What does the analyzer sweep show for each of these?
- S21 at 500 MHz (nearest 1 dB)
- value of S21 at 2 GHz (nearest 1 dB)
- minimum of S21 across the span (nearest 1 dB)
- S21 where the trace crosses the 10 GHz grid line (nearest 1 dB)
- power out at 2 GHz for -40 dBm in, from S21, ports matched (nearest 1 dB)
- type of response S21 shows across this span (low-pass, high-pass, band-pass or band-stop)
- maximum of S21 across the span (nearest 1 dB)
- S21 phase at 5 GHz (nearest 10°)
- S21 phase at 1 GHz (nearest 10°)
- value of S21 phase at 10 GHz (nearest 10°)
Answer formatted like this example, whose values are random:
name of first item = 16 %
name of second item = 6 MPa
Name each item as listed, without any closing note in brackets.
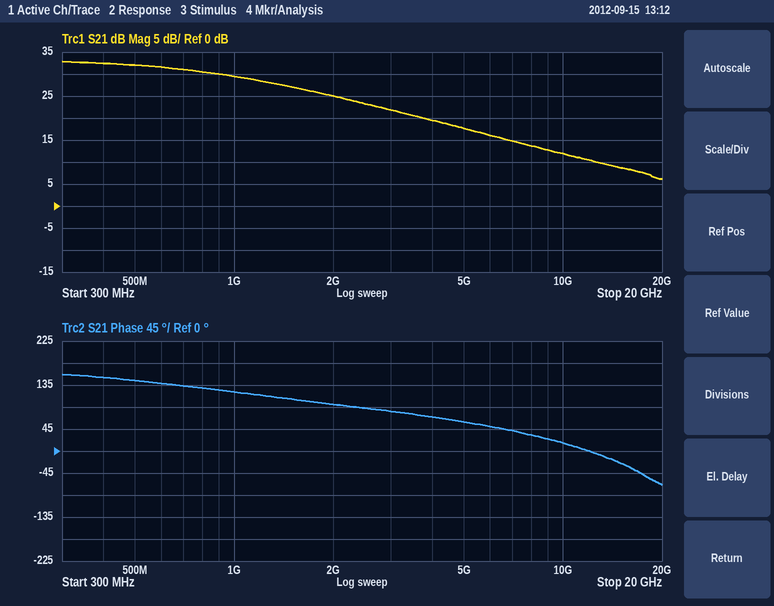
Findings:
S21 at 500 MHz = 32 dB
value of S21 at 2 GHz = 25 dB
minimum of S21 across the span = 6 dB
S21 where the trace crosses the 10 GHz grid line = 12 dB
power out at 2 GHz for -40 dBm in, from S21, ports matched = -15 dBm
type of response S21 shows across this span = low-pass
maximum of S21 across the span = 33 dB
S21 phase at 5 GHz = 60°
S21 phase at 1 GHz = 120°
value of S21 phase at 10 GHz = 20°
